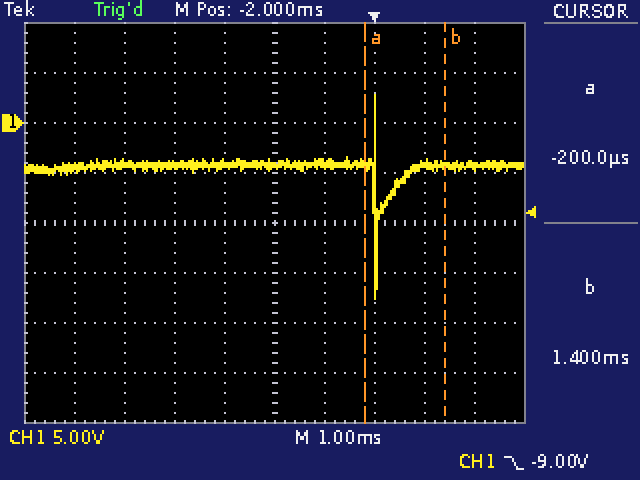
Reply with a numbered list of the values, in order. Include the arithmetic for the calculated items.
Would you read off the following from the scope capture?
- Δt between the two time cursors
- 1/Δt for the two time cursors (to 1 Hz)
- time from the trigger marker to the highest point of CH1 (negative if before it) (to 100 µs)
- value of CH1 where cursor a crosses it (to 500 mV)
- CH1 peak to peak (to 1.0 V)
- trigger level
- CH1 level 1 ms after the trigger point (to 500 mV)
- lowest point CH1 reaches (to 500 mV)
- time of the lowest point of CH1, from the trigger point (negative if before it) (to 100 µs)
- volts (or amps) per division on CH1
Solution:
1. 1.4 ms − (-200 µs) = 1.6 ms
2. 1 / 1.6 ms ≈ 625 Hz
3. 0.0 ms
4. -4.0 V
5. 20.0 V
6. -9.00 V
7. -4.0 V
8. -17.5 V
9. 0.0 ms
10. 5 V
